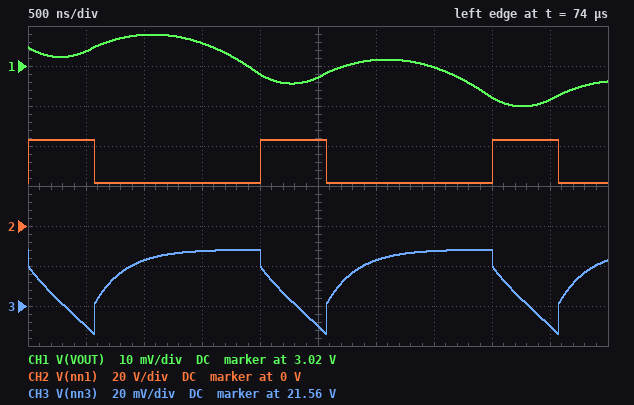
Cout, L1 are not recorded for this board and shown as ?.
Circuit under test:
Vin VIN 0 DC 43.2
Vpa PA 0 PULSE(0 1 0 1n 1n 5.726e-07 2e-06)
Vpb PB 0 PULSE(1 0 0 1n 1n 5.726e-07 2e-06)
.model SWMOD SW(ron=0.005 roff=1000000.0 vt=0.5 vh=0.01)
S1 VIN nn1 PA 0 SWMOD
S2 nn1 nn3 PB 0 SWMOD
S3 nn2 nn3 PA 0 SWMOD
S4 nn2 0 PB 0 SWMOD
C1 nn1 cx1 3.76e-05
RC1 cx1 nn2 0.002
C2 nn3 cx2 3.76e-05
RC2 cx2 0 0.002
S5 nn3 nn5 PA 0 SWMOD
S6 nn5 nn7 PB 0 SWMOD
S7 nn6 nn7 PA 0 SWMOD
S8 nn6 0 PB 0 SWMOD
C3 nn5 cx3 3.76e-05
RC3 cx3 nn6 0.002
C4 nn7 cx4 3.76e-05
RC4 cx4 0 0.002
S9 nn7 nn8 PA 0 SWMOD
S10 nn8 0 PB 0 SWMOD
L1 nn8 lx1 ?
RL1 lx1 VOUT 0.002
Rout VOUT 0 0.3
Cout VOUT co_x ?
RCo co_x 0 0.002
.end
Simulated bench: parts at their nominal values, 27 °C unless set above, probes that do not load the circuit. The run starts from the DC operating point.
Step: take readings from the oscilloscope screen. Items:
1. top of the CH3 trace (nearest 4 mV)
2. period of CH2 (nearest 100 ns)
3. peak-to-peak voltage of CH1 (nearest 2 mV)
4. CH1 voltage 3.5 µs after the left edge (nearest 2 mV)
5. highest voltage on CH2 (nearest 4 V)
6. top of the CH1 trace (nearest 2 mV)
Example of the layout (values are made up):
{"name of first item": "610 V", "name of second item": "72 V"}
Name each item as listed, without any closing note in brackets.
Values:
{"top of the CH3 trace": "21.588 V", "period of CH2": "2.0 µs", "peak-to-peak voltage of CH1": "18 mV", "CH1 voltage 3.5 µs after the left edge": "3.020 V", "highest voltage on CH2": "44 V", "top of the CH1 trace": "3.028 V"}
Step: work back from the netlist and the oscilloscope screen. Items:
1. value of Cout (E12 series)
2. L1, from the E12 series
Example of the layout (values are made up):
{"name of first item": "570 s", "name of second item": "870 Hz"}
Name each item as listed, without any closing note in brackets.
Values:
{"value of Cout": "27 µF", "L1, from the E12 series": "4.7 µH"}
